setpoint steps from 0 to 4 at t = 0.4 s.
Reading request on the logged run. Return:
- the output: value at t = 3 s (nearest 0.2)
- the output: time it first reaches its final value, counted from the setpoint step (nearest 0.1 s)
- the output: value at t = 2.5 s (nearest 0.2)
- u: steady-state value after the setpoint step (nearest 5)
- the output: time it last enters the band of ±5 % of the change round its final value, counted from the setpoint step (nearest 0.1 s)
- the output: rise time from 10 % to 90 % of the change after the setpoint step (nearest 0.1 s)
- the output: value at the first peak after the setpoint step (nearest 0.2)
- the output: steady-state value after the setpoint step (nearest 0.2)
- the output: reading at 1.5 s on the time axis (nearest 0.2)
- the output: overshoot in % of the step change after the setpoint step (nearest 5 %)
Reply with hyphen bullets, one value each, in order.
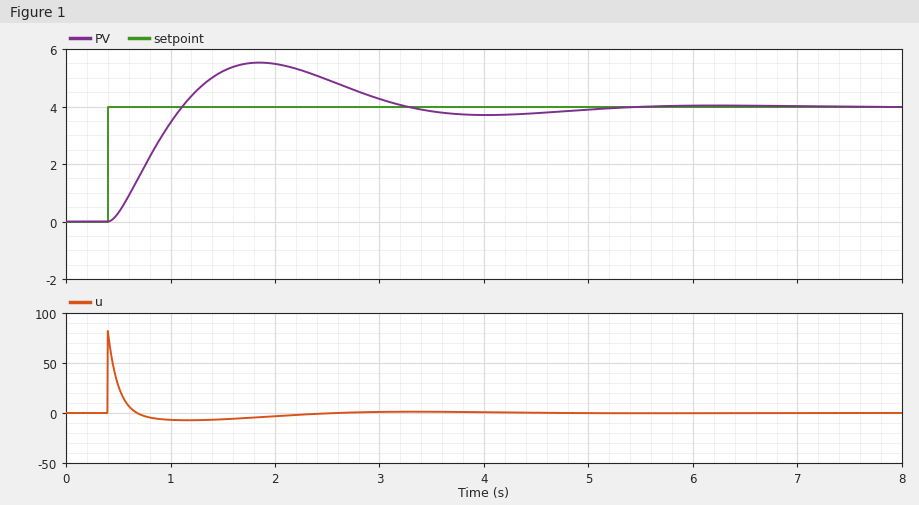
- 4.2
- 0.7 s
- 5.0
- 0
- 4.2 s
- 0.5 s
- 5.6
- 4.0
- 5.2
- 40 %
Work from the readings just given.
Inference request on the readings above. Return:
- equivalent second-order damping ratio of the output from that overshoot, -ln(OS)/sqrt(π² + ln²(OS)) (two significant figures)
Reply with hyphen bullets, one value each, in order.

- 0.28
